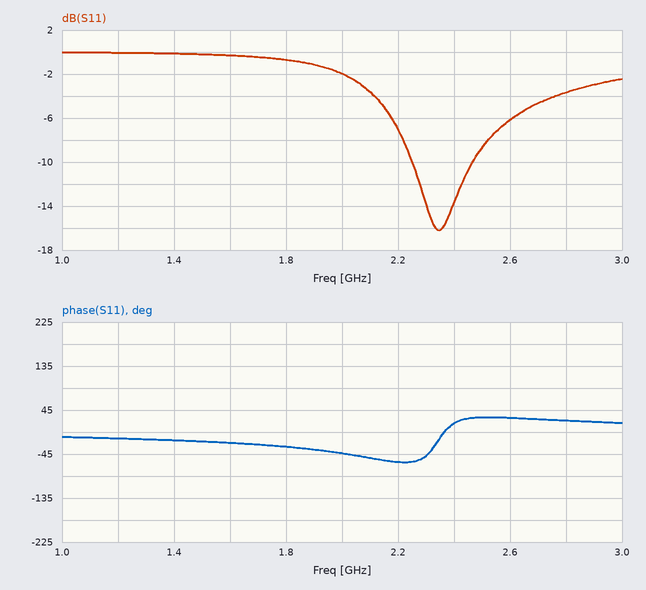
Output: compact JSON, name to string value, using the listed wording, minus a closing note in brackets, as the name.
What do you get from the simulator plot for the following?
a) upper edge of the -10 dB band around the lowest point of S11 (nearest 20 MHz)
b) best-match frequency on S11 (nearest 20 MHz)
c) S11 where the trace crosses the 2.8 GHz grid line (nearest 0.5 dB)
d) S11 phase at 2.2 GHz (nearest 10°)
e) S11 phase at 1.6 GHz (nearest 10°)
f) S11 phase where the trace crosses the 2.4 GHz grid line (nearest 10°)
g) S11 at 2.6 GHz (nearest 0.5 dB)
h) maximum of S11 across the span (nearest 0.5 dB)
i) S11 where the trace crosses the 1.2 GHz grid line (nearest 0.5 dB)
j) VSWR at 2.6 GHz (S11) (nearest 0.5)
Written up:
{"upper edge of the -10 dB band around the lowest point of S11": "2.46 GHz", "best-match frequency on S11": "2.34 GHz", "S11 where the trace crosses the 2.8 GHz grid line": "-3.5 dB", "S11 phase at 2.2 GHz": "-60°", "S11 phase at 1.6 GHz": "-20°", "S11 phase where the trace crosses the 2.4 GHz grid line": "20°", "S11 at 2.6 GHz": "-6.0 dB", "maximum of S11 across the span": "0.0 dB", "S11 where the trace crosses the 1.2 GHz grid line": "0.0 dB", "VSWR at 2.6 GHz (S11)": "3.0"}
